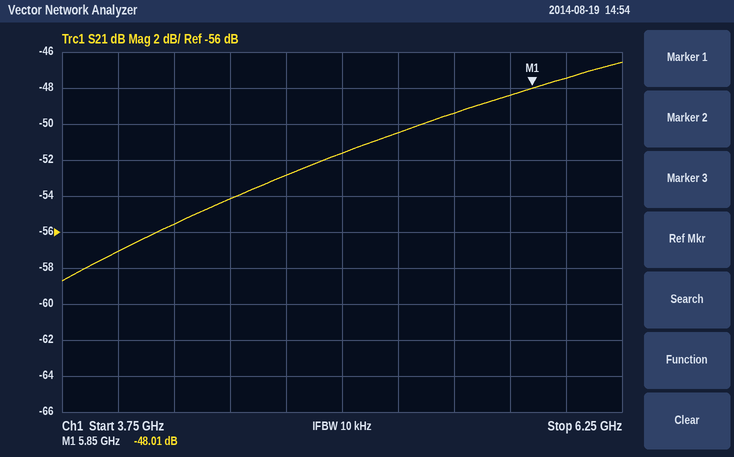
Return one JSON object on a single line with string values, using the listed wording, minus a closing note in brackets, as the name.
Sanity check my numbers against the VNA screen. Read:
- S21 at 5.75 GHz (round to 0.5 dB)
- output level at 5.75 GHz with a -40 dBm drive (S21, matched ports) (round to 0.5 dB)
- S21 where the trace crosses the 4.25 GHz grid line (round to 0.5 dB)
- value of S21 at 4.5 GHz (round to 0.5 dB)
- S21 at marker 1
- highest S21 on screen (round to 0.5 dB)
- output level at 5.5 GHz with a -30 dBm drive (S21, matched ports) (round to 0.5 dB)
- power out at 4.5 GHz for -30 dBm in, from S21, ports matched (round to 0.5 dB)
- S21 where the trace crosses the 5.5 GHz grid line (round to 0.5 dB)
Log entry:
{"S21 at 5.75 GHz": "-48.5 dB", "output level at 5.75 GHz with a -40 dBm drive (S21, matched ports)": "-88.5 dBm", "S21 where the trace crosses the 4.25 GHz grid line": "-55.5 dB", "value of S21 at 4.5 GHz": "-54.0 dB", "S21 at marker 1": "-48.01 dB", "highest S21 on screen": "-46.5 dB", "output level at 5.5 GHz with a -30 dBm drive (S21, matched ports)": "-79.5 dBm", "power out at 4.5 GHz for -30 dBm in, from S21, ports matched": "-84.0 dBm", "S21 where the trace crosses the 5.5 GHz grid line": "-49.5 dB"}
